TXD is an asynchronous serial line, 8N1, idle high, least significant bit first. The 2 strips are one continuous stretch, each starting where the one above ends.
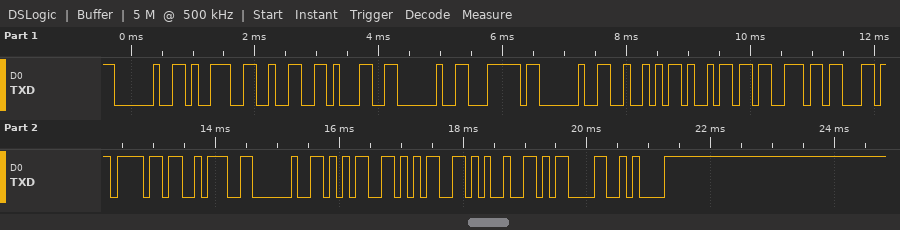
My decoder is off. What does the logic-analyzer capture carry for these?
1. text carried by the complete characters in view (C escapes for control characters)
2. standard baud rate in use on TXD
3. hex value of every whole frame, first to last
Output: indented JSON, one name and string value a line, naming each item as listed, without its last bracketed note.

{
  "text carried by the complete characters in view": "\" 921 | Risco: 55%\\r\\n\"",
  "standard baud rate in use on TXD": "9600 baud",
  "hex value of every whole frame, first to last": "20 39 32 31 20 7C 20 52 69 73 63 6F 3A 20 35 35 25 0D 0A"
}
